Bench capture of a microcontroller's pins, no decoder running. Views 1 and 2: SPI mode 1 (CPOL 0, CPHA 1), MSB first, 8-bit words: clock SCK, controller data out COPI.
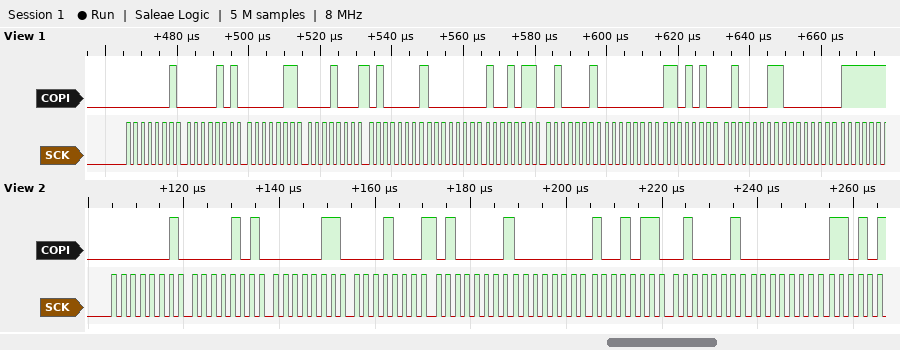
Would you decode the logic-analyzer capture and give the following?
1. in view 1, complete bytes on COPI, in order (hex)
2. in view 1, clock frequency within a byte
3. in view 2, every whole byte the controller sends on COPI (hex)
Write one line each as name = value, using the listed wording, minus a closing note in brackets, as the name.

in view 1, complete bytes on COPI, in order = 0x02 0x0A 0x06 0x11 0x41 0x00 0x96 0x42 0x00 0xD4 0x43 0x00
in view 1, clock frequency within a byte = 500 kHz
in view 2, every whole byte the controller sends on COPI = 02 0A 06 11 41 00 96 42 00
